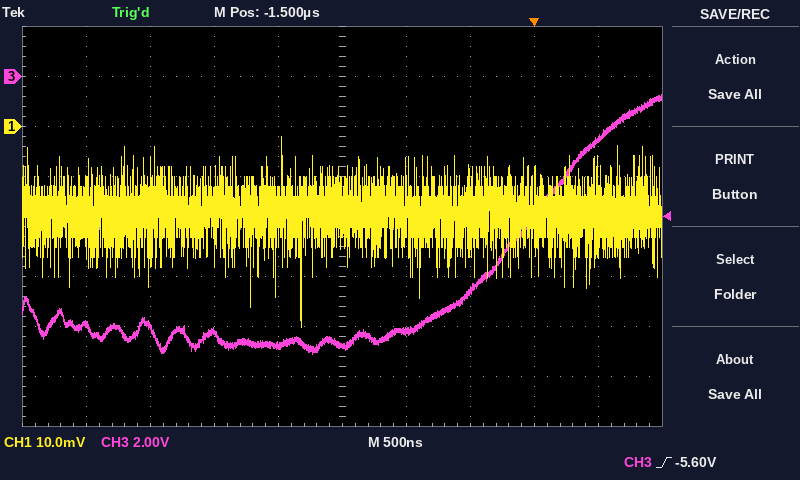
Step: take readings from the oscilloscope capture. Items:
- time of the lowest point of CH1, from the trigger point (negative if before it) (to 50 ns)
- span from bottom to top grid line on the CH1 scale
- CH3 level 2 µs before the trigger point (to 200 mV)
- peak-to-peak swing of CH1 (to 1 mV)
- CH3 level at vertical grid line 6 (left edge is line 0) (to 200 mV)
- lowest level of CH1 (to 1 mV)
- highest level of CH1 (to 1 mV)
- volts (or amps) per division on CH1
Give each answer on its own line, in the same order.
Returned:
-1.80 µs
80 mV
-10.8 V
38 mV
-10.2 V
-40 mV
-2 mV
10 mV
